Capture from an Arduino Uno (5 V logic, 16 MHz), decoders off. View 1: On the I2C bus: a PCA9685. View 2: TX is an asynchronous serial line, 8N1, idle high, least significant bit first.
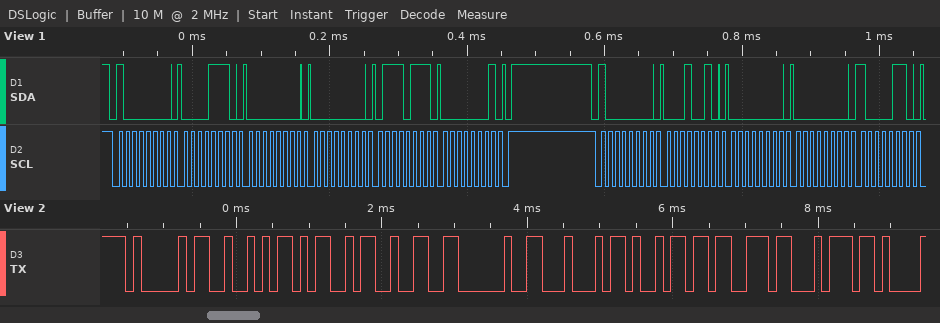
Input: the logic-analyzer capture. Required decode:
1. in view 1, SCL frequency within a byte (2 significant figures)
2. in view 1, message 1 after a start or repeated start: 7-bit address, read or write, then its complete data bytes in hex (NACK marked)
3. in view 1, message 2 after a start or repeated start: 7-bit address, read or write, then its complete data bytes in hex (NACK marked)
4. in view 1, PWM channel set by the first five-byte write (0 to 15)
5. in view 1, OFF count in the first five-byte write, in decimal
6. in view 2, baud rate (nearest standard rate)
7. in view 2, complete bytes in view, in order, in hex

100 kHz
0x40 write: 0E 00 00 77 01
0x40 write: 12 00 00 86
2
375
9600 baud
41 52 4D 32 20 44 69 73 74
